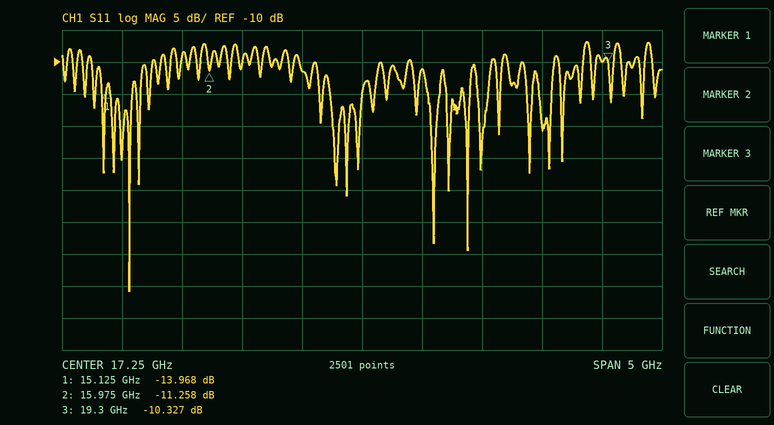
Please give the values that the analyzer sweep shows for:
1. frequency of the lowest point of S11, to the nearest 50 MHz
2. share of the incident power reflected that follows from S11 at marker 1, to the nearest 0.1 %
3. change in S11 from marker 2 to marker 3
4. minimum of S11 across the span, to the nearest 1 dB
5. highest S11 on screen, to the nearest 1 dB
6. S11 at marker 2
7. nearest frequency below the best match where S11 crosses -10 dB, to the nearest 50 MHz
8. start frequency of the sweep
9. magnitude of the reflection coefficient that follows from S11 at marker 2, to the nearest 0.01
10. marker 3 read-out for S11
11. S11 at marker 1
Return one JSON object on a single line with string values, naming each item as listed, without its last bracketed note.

{"frequency of the lowest point of S11, to the nearest 50 MHz": "15.30 GHz", "share of the incident power reflected that follows from S11 at marker 1, to the nearest 0.1 %": "4.0 %", "change in S11 from marker 2 to marker 3": "0.931 dB", "minimum of S11 across the span, to the nearest 1 dB": "-46 dB", "highest S11 on screen, to the nearest 1 dB": "-7 dB", "S11 at marker 2": "-11.258 dB", "nearest frequency below the best match where S11 crosses -10 dB, to the nearest 50 MHz": "15.00 GHz", "start frequency of the sweep": "14.75 GHz", "magnitude of the reflection coefficient that follows from S11 at marker 2, to the nearest 0.01": "0.27", "marker 3 read-out for S11": "-10.327 dB", "S11 at marker 1": "-13.968 dB"}
